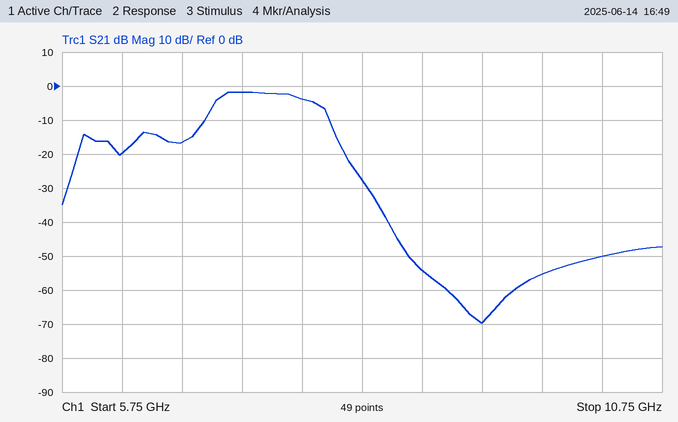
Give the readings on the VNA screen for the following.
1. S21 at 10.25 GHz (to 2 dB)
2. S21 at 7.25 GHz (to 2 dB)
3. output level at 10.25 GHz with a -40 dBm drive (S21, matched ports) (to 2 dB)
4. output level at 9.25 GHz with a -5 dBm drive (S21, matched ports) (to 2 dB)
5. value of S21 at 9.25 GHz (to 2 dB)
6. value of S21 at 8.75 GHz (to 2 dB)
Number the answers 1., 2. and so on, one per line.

1. -50 dB
2. -2 dB
3. -90 dBm
4. -74 dBm
5. -70 dB
6. -54 dB
